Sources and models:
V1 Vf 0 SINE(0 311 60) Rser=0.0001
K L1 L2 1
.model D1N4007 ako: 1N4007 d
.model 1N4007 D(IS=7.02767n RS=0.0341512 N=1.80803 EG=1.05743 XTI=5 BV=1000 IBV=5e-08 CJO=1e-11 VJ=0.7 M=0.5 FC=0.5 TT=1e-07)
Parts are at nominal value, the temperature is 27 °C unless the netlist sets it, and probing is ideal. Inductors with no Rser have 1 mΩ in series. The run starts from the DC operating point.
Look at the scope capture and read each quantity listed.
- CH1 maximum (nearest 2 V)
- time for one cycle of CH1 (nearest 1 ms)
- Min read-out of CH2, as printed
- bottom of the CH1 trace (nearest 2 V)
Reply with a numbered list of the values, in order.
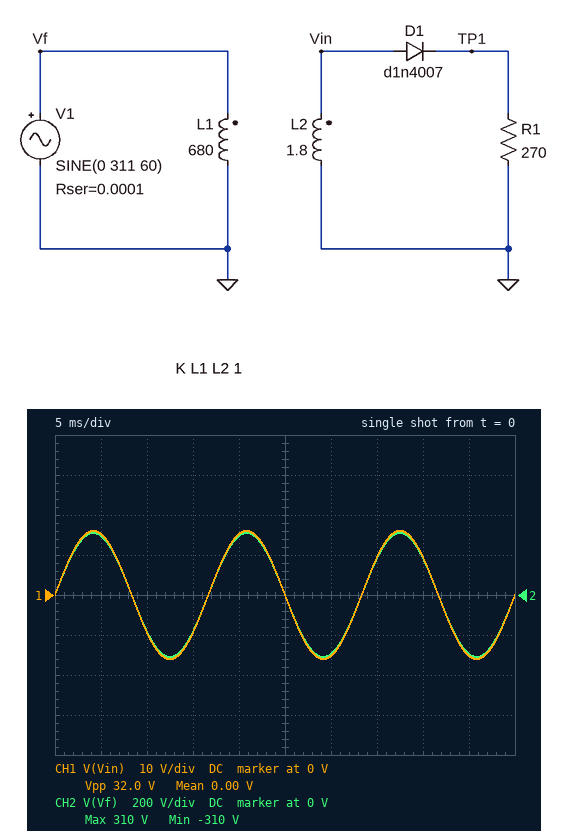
1. 16 V
2. 17 ms
3. -310 V
4. -16 V
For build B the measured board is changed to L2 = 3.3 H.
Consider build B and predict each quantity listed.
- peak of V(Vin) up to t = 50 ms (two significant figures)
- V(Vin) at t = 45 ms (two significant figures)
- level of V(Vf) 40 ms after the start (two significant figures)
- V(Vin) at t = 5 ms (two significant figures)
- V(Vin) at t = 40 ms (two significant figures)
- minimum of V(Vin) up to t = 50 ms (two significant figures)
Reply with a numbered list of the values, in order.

1. 22 V
2. -21 V
3. 180 V
4. 21 V
5. 13 V
6. -22 V
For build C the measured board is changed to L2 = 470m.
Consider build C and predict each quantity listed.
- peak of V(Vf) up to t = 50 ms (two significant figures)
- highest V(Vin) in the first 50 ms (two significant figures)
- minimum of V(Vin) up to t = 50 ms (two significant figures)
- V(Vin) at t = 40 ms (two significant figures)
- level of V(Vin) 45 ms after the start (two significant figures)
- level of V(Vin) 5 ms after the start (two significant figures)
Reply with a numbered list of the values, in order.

1. 310 V
2. 8.2 V
3. -8.2 V
4. 4.8 V
5. -7.8 V
6. 7.8 V
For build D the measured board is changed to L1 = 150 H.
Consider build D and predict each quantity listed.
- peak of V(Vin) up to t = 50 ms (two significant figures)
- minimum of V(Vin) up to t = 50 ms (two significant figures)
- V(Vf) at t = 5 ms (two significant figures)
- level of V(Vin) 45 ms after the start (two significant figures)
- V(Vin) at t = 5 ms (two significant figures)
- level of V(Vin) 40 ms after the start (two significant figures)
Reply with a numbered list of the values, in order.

1. 34 V
2. -34 V
3. 300 V
4. -32 V
5. 32 V
6. 20 V
